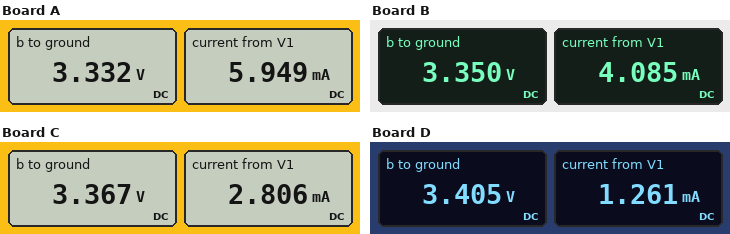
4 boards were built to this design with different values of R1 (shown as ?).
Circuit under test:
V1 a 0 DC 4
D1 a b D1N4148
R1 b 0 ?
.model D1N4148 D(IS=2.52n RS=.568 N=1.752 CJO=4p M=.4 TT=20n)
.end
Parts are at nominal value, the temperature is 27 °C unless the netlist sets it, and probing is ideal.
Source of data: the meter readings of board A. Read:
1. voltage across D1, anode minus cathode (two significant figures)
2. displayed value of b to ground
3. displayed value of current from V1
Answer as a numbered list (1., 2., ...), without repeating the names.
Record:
1. 670 mV
2. 3.332 V
3. 5.949 mA
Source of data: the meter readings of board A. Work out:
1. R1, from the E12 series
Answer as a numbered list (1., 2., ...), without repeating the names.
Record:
1. 560 Ω
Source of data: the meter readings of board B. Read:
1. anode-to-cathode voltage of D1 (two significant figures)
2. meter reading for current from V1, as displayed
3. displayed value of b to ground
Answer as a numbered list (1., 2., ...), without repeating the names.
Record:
1. 650 mV
2. 4.085 mA
3. 3.350 V
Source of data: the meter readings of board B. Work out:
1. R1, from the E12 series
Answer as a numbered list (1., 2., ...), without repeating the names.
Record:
1. 820 Ω
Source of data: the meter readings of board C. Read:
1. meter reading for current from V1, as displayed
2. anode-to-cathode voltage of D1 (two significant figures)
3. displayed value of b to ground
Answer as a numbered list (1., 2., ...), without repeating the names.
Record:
1. 2.806 mA
2. 630 mV
3. 3.367 V
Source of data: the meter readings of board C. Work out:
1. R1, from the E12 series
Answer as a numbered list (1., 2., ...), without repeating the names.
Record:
1. 1.2 kΩ
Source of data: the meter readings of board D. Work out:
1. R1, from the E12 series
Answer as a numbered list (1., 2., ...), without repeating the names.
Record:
1. 2.7 kΩ
